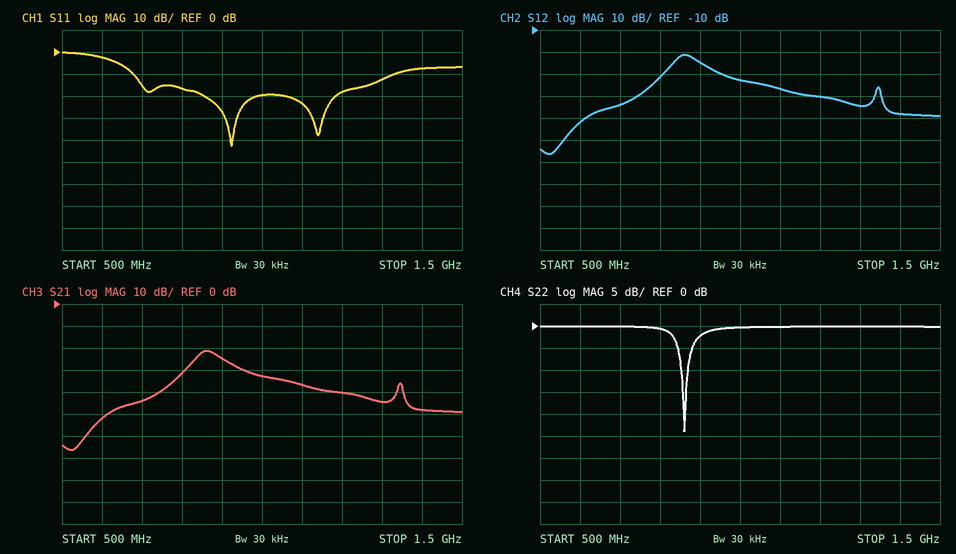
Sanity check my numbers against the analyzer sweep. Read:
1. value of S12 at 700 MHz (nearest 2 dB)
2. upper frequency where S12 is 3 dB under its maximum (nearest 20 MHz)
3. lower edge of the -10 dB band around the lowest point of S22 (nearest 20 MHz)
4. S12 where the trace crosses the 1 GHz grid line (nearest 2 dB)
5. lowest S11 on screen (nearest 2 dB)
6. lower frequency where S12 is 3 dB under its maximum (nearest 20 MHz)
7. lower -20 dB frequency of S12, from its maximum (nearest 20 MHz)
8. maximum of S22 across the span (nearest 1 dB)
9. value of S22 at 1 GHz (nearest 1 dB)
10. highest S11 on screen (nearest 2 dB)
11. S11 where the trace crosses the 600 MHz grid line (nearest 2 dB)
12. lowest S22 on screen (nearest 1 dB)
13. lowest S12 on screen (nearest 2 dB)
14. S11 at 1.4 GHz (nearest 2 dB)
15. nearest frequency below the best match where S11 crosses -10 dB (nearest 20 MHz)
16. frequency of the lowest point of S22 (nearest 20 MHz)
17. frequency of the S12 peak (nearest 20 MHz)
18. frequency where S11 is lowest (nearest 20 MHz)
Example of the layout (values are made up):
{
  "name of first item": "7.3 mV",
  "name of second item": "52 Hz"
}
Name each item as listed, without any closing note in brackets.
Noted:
{
  "value of S12 at 700 MHz": "-44 dB",
  "upper frequency where S12 is 3 dB under its maximum": "900 MHz",
  "lower edge of the -10 dB band around the lowest point of S22": "860 MHz",
  "S12 where the trace crosses the 1 GHz grid line": "-32 dB",
  "lowest S11 on screen": "-42 dB",
  "lower frequency where S12 is 3 dB under its maximum": "840 MHz",
  "lower -20 dB frequency of S12, from its maximum": "740 MHz",
  "maximum of S22 across the span": "0 dB",
  "value of S22 at 1 GHz": "0 dB",
  "highest S11 on screen": "0 dB",
  "S11 where the trace crosses the 600 MHz grid line": "-2 dB",
  "lowest S22 on screen": "-24 dB",
  "lowest S12 on screen": "-66 dB",
  "S11 at 1.4 GHz": "-8 dB",
  "nearest frequency below the best match where S11 crosses -10 dB": "680 MHz",
  "frequency of the lowest point of S22": "860 MHz",
  "frequency of the S12 peak": "860 MHz",
  "frequency where S11 is lowest": "920 MHz"
}
